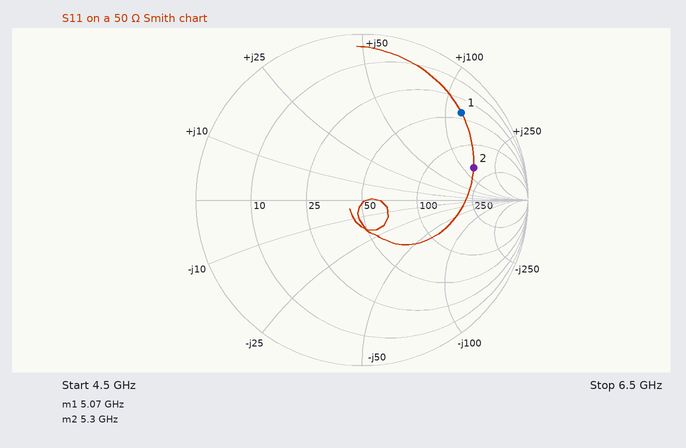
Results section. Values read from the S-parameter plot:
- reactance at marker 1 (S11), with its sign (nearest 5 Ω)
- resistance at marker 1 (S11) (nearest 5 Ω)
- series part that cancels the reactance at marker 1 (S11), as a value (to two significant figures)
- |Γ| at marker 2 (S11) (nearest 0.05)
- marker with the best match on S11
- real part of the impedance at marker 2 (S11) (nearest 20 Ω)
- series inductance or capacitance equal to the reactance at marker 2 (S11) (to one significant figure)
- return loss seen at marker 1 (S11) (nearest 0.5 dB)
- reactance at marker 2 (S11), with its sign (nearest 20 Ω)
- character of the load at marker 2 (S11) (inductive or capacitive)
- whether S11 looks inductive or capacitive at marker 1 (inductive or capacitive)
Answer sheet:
+120 Ω
40 Ω
260 fF
0.70
marker 2
180 Ω
4 nH
2.0 dB
+140 Ω
inductive
inductive
